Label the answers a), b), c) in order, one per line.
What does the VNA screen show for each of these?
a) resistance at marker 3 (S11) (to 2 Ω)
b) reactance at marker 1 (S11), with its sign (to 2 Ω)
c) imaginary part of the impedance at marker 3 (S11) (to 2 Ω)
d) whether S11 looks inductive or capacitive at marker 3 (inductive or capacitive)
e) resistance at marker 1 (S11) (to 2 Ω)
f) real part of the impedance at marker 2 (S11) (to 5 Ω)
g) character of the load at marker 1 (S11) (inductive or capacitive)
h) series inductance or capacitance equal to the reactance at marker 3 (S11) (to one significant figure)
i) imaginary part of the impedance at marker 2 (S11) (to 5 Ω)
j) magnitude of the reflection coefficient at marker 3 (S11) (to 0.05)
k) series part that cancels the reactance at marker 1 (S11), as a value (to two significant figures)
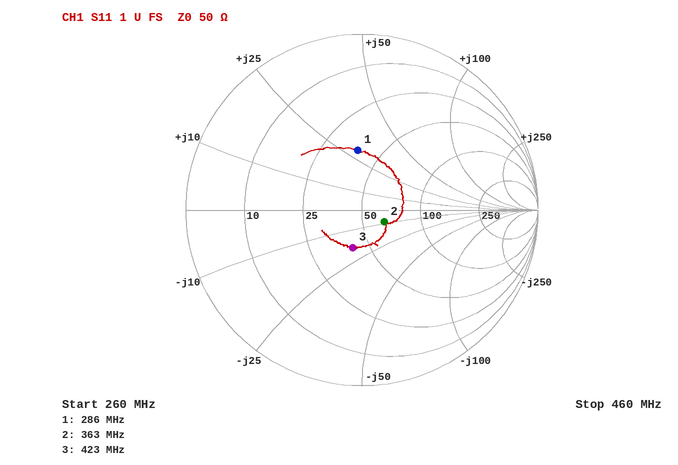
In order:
a) 42 Ω
b) +30 Ω
c) -18 Ω
d) capacitive
e) 38 Ω
f) 65 Ω
g) inductive
h) 20 pF
i) -10 Ω
j) 0.20
k) 19 pF
